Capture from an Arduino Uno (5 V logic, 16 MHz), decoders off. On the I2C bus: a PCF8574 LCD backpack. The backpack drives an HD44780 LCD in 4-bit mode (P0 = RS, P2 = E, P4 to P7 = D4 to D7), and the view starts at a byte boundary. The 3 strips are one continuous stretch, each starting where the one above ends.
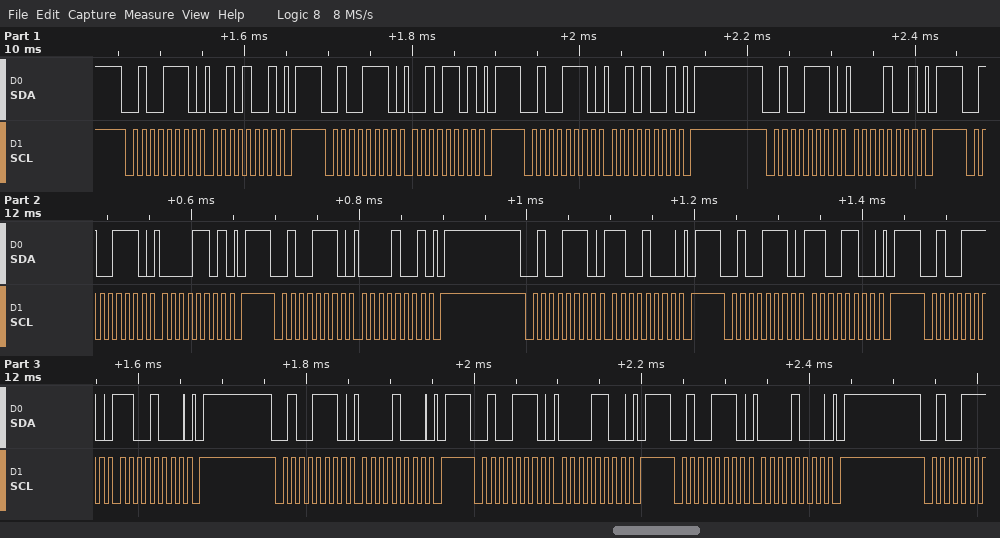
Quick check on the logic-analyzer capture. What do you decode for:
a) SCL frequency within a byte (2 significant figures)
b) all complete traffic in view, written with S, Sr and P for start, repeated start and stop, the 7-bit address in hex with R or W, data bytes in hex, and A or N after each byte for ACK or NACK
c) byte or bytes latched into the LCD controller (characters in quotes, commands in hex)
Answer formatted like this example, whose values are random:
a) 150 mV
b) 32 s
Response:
a) 100 kHz
b) S 27W A 29 A P S 27W A 2D A P S 27W A 29 A P S 27W A 09 A P S 27W A 0D A P S 27W A 09 A P S 27W A C8 A P S 27W A CC A P S 27W A C8 A P S 27W A 08 A P S 27W A 0C A P S 27W A 08 A P
c) ' ' 0xC0
